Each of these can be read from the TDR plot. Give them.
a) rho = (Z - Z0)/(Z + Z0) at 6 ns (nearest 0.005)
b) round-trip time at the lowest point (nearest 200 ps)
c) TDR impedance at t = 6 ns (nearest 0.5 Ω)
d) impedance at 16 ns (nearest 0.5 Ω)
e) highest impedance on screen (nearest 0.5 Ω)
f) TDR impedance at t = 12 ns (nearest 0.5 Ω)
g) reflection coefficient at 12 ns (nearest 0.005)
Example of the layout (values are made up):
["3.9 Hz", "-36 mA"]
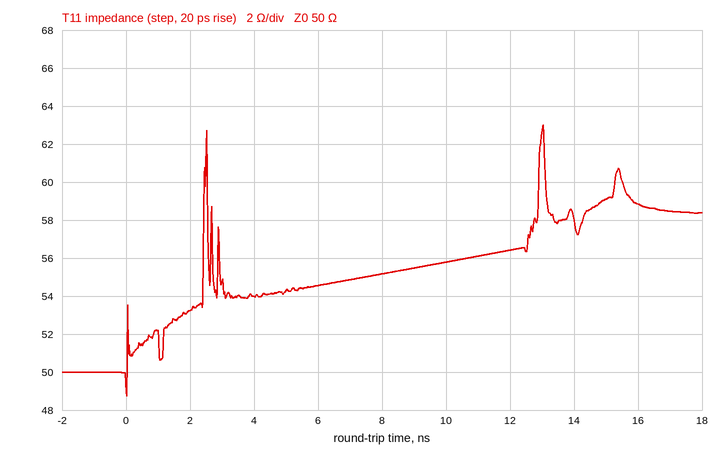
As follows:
["+0.045", "0.0 ns", "54.5 Ω", "59.0 Ω", "63.0 Ω", "56.5 Ω", "+0.060"]
